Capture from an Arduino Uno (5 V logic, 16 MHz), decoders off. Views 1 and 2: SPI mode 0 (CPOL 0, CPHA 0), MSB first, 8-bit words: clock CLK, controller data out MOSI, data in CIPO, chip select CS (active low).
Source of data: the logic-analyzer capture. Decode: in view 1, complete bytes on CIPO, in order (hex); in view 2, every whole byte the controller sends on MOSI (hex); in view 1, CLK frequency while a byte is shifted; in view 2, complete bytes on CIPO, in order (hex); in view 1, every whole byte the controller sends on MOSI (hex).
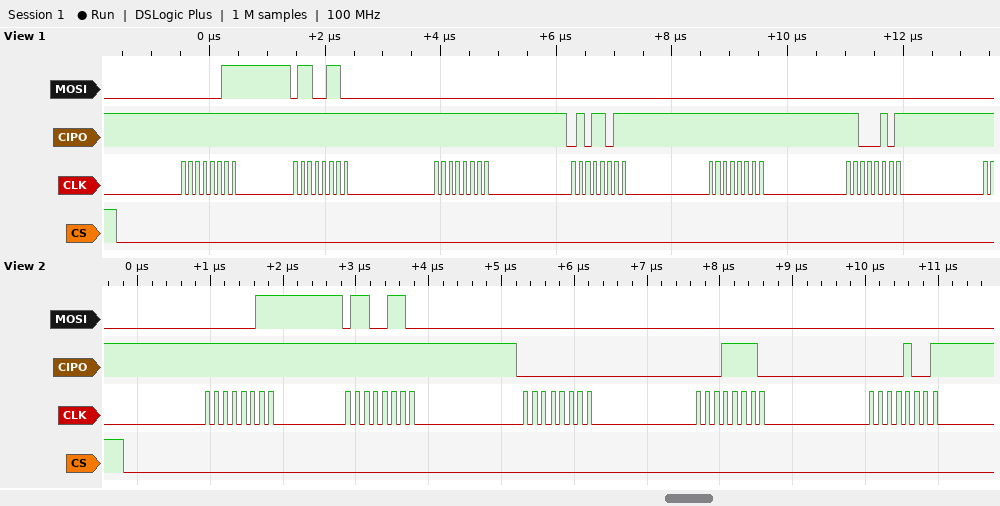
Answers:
FF FF FF 5B FF C5
0x03 0x66 0x00 0x00 0x00
8 MHz
0xFF 0xFF 0x00 0x1E 0x09
03 66 00 00 00 00
